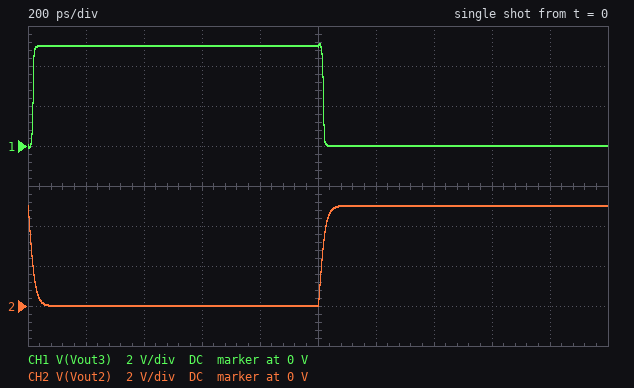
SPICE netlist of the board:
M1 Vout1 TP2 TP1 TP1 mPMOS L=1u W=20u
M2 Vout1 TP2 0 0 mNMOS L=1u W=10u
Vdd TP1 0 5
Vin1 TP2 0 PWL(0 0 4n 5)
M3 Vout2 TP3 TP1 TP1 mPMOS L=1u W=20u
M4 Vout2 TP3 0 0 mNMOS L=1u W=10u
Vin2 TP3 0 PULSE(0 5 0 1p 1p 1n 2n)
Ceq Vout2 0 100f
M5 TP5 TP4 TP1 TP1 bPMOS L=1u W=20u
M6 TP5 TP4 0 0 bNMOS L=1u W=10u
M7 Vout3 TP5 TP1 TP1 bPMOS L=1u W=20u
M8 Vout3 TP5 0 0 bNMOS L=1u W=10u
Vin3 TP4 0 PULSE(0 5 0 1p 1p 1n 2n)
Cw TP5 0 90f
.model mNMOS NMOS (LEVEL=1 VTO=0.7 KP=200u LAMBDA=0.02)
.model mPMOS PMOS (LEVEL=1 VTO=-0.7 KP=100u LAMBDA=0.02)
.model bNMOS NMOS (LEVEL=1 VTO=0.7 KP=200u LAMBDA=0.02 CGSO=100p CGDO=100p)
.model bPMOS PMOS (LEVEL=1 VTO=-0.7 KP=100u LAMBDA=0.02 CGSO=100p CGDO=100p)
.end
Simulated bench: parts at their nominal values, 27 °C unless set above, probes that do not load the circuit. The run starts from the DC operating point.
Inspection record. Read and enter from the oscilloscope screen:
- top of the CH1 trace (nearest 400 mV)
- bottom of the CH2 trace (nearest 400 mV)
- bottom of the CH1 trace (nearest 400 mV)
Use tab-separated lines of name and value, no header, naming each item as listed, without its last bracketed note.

top of the CH1 trace	5.2 V
bottom of the CH2 trace	0 V
bottom of the CH1 trace	0 V
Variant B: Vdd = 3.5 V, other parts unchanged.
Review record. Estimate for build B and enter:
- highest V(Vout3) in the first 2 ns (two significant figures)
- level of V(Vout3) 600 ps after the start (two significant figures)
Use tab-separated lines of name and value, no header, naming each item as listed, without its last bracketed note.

highest V(Vout3) in the first 2 ns	3.6 V
level of V(Vout3) 600 ps after the start	3.5 V
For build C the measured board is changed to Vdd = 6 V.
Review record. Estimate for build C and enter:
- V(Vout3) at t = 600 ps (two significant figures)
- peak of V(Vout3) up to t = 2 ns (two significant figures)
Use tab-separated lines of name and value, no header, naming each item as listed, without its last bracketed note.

V(Vout3) at t = 600 ps	6.0 V
peak of V(Vout3) up to t = 2 ns	6.1 V
